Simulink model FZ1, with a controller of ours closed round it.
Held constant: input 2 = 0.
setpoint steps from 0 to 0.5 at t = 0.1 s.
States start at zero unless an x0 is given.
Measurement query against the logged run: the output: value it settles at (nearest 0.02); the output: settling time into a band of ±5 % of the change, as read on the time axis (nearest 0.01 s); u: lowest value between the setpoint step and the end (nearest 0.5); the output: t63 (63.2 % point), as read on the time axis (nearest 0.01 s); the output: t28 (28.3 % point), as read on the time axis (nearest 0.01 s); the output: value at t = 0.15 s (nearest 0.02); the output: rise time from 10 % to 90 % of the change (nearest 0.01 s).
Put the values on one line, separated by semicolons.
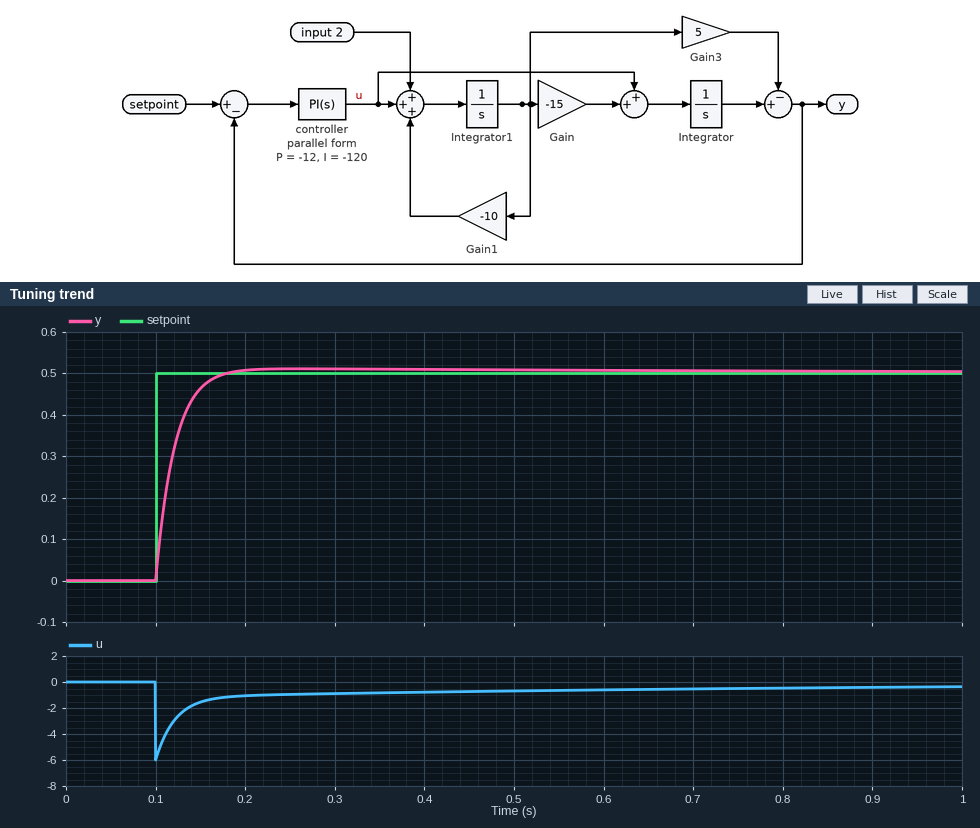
0.50; 0.16 s; -6.0; 0.12 s; 0.11 s; 0.46; 0.04 s
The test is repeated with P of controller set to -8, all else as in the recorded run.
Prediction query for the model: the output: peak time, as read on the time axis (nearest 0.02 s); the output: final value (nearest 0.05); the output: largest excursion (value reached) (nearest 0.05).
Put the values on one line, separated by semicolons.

0.22 s; 0.50; 0.55
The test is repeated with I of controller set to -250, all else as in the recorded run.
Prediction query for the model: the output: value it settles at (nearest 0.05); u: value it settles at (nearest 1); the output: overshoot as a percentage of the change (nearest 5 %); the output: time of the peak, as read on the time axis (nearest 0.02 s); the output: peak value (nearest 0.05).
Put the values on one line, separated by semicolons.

0.50; 0; 10 %; 0.18 s; 0.55
